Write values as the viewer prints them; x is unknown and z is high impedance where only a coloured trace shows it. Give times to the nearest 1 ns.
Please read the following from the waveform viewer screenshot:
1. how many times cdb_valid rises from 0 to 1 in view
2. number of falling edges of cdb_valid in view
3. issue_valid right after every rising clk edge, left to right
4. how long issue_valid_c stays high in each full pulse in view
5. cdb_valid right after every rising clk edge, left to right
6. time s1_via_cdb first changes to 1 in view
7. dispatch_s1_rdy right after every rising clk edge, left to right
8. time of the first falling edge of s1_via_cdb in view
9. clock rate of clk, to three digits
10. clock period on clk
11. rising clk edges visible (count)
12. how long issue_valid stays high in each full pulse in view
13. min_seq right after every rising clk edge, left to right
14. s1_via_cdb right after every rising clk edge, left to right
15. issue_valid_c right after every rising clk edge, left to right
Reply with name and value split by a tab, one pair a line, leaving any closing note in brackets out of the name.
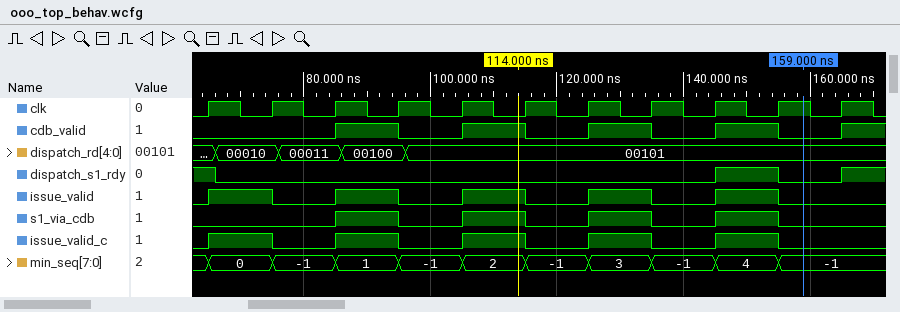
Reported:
how many times cdb_valid rises from 0 to 1 in view	5
number of falling edges of cdb_valid in view	4
issue_valid right after every rising clk edge, left to right	1 0 1 0 1 0 1 0 1 0 0
how long issue_valid_c stays high in each full pulse in view	10 ns, 10 ns, 10 ns, 10 ns, 10 ns
cdb_valid right after every rising clk edge, left to right	0 0 1 0 1 0 1 0 1 0 1
time s1_via_cdb first changes to 1 in view	85 ns
dispatch_s1_rdy right after every rising clk edge, left to right	1 0 0 0 0 0 0 0 1 0 1
time of the first falling edge of s1_via_cdb in view	95 ns
clock rate of clk, to three digits	100 MHz
clock period on clk	10 ns
rising clk edges visible	11
how long issue_valid stays high in each full pulse in view	10 ns, 10 ns, 10 ns, 10 ns, 10 ns
min_seq right after every rising clk edge, left to right	0, -1, 1, -1, 2, -1, 3, -1, 4, -1, -1
s1_via_cdb right after every rising clk edge, left to right	0 0 1 0 1 0 1 0 1 0 0
issue_valid_c right after every rising clk edge, left to right	1 0 1 0 1 0 1 0 1 0 0
